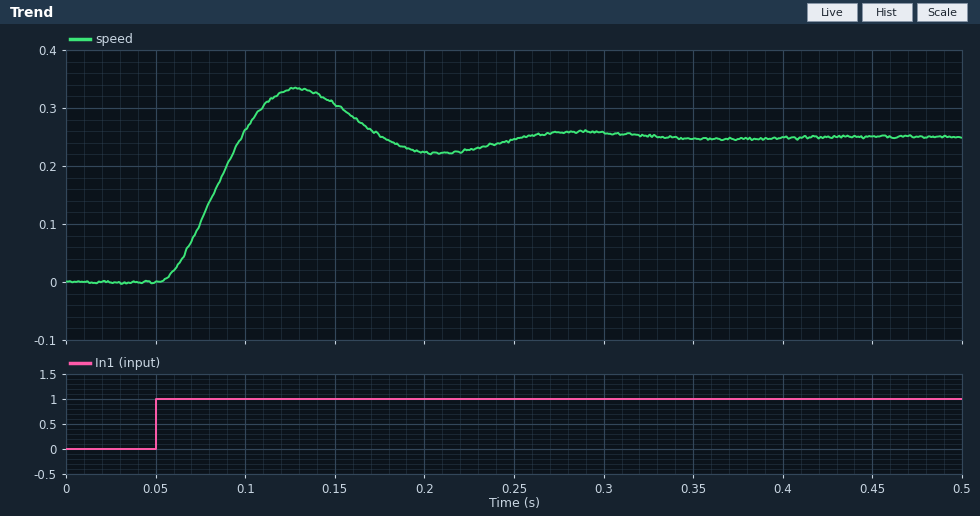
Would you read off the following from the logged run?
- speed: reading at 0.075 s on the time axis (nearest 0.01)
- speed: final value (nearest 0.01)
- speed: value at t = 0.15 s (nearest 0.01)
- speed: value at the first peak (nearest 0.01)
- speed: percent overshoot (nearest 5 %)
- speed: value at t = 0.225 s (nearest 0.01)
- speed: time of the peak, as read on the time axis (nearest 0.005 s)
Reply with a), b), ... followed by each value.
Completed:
a) 0.10
b) 0.25
c) 0.31
d) 0.33
e) 35 %
f) 0.23
g) 0.130 s
